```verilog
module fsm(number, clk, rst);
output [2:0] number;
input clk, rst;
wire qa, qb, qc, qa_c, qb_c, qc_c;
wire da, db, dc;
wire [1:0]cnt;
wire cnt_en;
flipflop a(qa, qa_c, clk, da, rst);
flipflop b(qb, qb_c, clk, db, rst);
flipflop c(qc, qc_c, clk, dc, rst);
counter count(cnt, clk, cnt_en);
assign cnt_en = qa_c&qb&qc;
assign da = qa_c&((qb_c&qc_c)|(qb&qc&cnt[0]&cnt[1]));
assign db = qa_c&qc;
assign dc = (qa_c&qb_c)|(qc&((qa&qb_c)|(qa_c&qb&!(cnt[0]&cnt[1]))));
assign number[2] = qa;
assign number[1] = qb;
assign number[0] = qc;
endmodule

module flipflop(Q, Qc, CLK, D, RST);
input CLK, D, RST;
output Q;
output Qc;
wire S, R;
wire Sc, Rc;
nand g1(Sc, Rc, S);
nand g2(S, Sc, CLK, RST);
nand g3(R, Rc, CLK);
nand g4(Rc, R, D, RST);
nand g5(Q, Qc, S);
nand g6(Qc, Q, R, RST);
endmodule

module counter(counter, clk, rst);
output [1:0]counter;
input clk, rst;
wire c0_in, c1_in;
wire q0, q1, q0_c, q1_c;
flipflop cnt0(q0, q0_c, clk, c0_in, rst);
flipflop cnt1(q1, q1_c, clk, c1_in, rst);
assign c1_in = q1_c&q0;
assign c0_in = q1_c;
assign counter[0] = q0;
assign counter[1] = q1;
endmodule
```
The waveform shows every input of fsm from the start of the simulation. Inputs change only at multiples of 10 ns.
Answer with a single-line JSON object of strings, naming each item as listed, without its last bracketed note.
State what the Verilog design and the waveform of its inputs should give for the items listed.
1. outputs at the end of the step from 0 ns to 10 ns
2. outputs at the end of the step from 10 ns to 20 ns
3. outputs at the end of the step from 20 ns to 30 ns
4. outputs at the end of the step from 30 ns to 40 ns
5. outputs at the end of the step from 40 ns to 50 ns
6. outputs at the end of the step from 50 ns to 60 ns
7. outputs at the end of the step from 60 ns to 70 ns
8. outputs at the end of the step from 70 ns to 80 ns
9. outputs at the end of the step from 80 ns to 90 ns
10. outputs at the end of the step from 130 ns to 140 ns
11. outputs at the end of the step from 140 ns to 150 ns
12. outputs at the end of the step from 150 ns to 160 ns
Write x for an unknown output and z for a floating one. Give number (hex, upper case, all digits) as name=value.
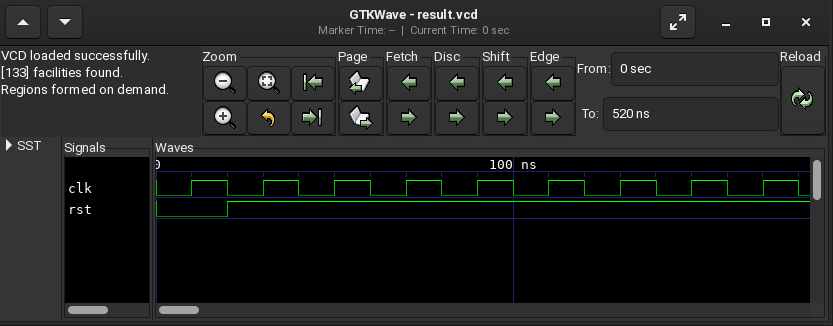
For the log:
{"outputs at the end of the step from 0 ns to 10 ns": "number=0", "outputs at the end of the step from 10 ns to 20 ns": "number=0", "outputs at the end of the step from 20 ns to 30 ns": "number=0", "outputs at the end of the step from 30 ns to 40 ns": "number=5", "outputs at the end of the step from 40 ns to 50 ns": "number=5", "outputs at the end of the step from 50 ns to 60 ns": "number=1", "outputs at the end of the step from 60 ns to 70 ns": "number=1", "outputs at the end of the step from 70 ns to 80 ns": "number=3", "outputs at the end of the step from 80 ns to 90 ns": "number=3", "outputs at the end of the step from 130 ns to 140 ns": "number=6", "outputs at the end of the step from 140 ns to 150 ns": "number=6", "outputs at the end of the step from 150 ns to 160 ns": "number=0"}
